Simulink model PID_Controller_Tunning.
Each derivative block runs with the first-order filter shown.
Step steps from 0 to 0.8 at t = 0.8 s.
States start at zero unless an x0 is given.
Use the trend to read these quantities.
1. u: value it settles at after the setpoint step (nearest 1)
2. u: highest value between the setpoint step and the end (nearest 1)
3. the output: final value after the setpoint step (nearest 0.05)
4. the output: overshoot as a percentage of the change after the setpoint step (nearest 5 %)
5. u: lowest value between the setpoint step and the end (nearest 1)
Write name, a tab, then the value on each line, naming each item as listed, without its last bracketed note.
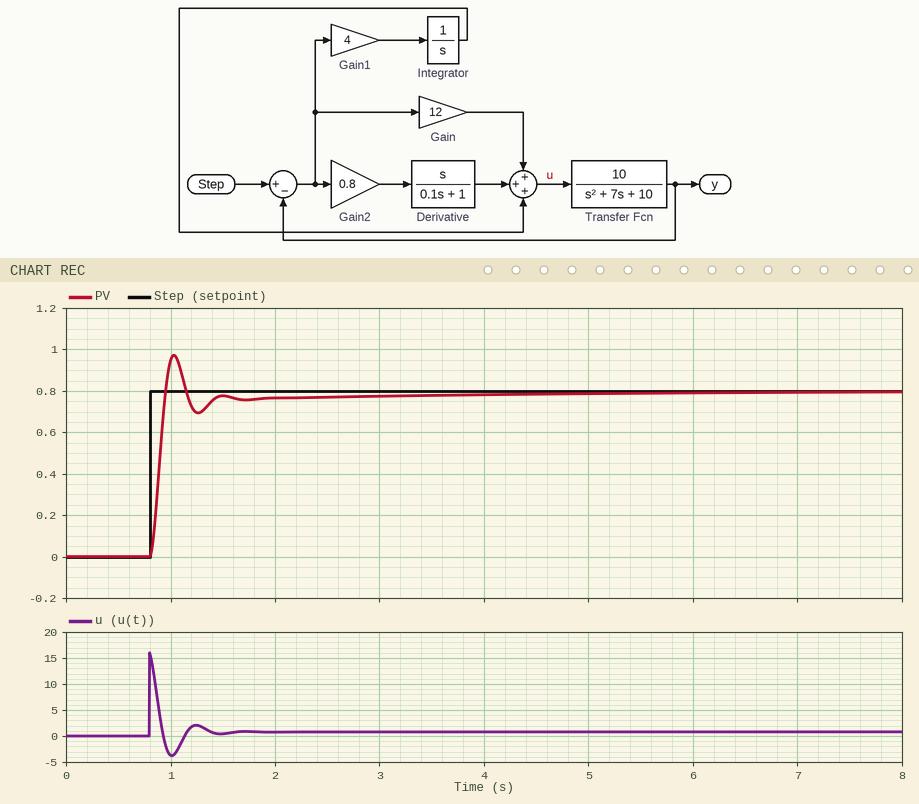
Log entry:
u: value it settles at after the setpoint step	1
u: highest value between the setpoint step and the end	16
the output: final value after the setpoint step	0.80
the output: overshoot as a percentage of the change after the setpoint step	20 %
u: lowest value between the setpoint step and the end	-4
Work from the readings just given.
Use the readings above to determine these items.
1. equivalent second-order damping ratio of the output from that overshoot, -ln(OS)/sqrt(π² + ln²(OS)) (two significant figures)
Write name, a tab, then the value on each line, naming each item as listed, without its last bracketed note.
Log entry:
equivalent second-order damping ratio of the output from that overshoot, -ln(OS)/sqrt(π² + ln²(OS))	0.46
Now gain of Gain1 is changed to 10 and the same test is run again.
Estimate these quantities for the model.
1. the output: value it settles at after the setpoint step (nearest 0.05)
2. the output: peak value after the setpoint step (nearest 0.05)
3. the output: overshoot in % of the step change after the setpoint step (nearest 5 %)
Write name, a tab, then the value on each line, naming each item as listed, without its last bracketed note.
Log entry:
the output: value it settles at after the setpoint step	0.80
the output: peak value after the setpoint step	1.00
the output: overshoot in % of the step change after the setpoint step	25 %
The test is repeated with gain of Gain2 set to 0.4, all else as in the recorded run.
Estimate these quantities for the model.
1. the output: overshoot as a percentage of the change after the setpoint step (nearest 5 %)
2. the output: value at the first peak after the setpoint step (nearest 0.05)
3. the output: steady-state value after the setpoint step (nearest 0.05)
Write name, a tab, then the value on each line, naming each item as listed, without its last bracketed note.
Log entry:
the output: overshoot as a percentage of the change after the setpoint step	25 %
the output: value at the first peak after the setpoint step	1.00
the output: steady-state value after the setpoint step	0.80
